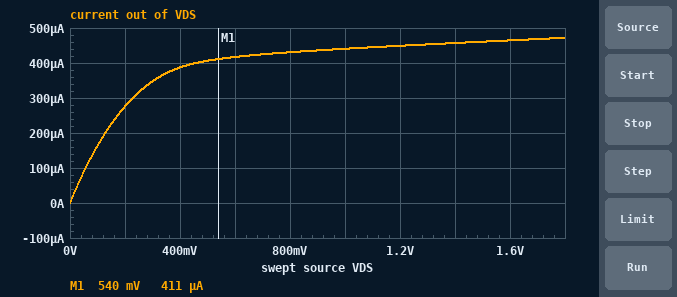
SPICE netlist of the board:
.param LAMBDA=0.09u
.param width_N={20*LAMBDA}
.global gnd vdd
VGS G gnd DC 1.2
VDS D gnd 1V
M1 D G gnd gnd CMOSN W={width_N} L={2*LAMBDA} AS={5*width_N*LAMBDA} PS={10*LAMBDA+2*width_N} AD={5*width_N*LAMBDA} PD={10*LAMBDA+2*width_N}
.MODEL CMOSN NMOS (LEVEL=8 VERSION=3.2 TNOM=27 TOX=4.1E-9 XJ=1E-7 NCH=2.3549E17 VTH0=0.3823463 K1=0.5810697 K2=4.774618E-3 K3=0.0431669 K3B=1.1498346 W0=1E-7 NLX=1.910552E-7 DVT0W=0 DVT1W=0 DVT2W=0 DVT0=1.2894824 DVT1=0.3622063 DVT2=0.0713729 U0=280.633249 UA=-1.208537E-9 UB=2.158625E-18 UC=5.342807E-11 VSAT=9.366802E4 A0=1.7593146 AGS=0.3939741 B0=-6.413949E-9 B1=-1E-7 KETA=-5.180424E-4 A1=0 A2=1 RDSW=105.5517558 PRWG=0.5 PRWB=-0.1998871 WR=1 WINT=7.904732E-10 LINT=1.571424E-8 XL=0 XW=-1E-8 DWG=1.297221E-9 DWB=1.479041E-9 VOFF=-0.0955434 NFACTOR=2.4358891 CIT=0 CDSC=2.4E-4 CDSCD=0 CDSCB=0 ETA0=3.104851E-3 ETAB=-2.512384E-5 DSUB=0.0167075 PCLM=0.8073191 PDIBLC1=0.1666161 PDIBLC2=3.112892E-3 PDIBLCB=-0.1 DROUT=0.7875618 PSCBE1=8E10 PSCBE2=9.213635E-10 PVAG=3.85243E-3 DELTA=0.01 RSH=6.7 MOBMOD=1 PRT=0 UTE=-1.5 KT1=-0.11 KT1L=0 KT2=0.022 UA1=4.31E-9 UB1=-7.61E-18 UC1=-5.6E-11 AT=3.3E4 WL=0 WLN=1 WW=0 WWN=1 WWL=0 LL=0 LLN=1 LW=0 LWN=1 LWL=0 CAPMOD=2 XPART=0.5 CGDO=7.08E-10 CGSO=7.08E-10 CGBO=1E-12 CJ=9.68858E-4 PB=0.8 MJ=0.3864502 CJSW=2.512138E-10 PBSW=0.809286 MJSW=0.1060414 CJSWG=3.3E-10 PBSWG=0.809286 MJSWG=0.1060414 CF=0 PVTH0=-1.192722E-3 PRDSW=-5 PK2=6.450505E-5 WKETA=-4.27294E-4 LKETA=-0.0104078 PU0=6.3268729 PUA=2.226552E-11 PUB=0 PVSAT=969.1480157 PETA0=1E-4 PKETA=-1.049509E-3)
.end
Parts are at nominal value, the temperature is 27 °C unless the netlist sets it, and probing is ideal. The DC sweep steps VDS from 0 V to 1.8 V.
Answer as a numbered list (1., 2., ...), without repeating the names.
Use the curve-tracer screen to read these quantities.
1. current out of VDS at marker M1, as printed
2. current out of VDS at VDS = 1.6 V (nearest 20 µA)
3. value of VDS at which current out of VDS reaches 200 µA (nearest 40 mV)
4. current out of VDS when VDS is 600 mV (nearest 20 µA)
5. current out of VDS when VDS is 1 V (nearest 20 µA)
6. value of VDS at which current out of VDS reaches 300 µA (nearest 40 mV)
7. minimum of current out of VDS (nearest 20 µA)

1. 411 µA
2. 460 µA
3. 120 mV
4. 420 µA
5. 440 µA
6. 240 mV
7. 0 A
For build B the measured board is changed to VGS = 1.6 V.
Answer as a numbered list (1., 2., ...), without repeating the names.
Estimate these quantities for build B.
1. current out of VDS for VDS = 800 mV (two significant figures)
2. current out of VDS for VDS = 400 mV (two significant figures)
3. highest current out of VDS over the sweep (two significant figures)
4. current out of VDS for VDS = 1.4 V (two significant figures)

1. 770 µA
2. 630 µA
3. 830 µA
4. 810 µA
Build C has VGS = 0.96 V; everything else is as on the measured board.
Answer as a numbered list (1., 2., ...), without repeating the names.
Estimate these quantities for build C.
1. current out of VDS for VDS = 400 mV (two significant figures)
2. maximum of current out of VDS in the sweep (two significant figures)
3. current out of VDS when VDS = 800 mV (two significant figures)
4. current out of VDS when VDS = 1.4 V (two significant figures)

1. 220 µA
2. 270 µA
3. 240 µA
4. 260 µA
